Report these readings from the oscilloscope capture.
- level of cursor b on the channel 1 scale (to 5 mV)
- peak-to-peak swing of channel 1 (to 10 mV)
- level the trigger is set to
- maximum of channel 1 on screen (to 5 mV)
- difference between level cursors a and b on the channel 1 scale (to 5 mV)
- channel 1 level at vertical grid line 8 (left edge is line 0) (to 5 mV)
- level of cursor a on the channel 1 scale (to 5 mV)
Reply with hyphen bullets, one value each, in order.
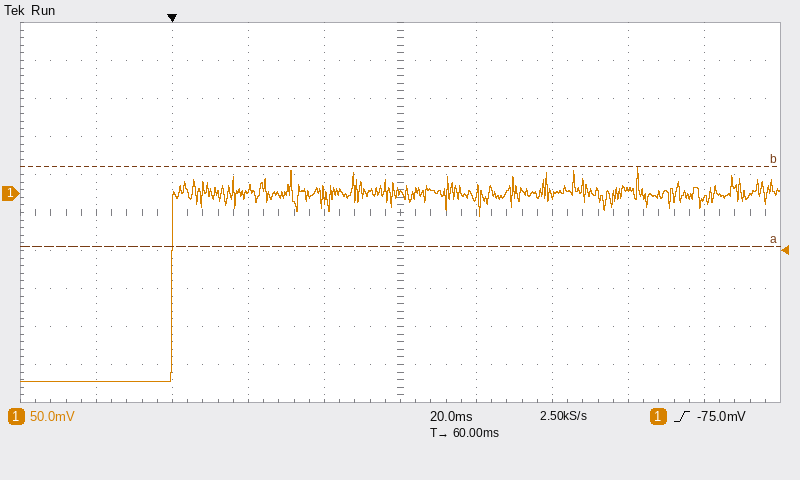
- 35 mV
- 280 mV
- -75.0 mV
- 35 mV
- 105 mV
- 5 mV
- -70 mV
